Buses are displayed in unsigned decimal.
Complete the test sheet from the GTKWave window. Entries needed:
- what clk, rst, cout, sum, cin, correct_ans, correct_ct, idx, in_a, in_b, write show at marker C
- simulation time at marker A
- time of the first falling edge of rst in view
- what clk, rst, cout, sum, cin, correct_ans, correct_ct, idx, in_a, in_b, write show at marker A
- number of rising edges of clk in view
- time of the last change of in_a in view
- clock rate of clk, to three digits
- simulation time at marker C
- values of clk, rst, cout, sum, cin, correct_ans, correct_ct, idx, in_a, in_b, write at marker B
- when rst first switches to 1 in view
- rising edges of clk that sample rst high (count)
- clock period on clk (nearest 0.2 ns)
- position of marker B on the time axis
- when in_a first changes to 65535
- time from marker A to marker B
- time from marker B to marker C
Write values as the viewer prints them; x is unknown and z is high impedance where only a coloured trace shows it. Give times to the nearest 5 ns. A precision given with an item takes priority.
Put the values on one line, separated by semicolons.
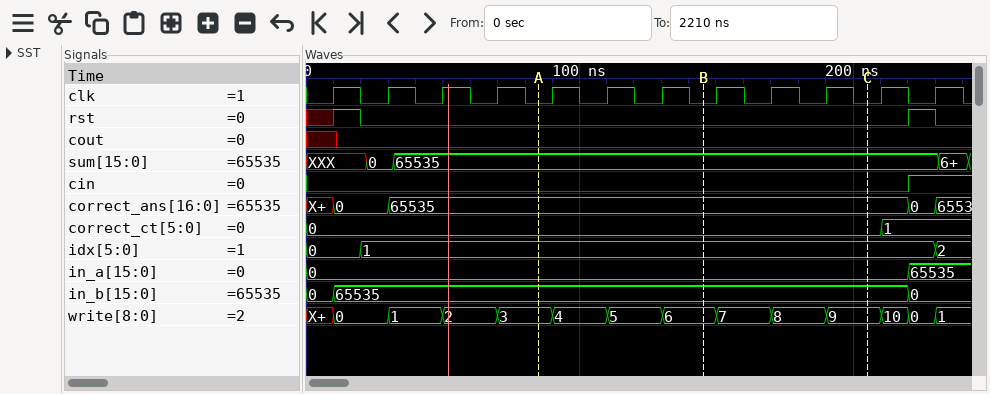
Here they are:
clk=0, rst=0, cout=0, sum=65535, cin=0, correct_ans=65535, correct_ct=0, idx=1, in_a=0, in_b=65535, write=9; 85 ns; 20 ns; clk=0, rst=0, cout=0, sum=65535, cin=0, correct_ans=65535, correct_ct=0, idx=1, in_a=0, in_b=65535, write=3; 12; 220 ns; 50.0 MHz; 205 ns; clk=0, rst=0, cout=0, sum=65535, cin=0, correct_ans=65535, correct_ct=0, idx=1, in_a=0, in_b=65535, write=6; 10 ns; 1; 20 ns; 145 ns; 220 ns; 60 ns; 60 ns
